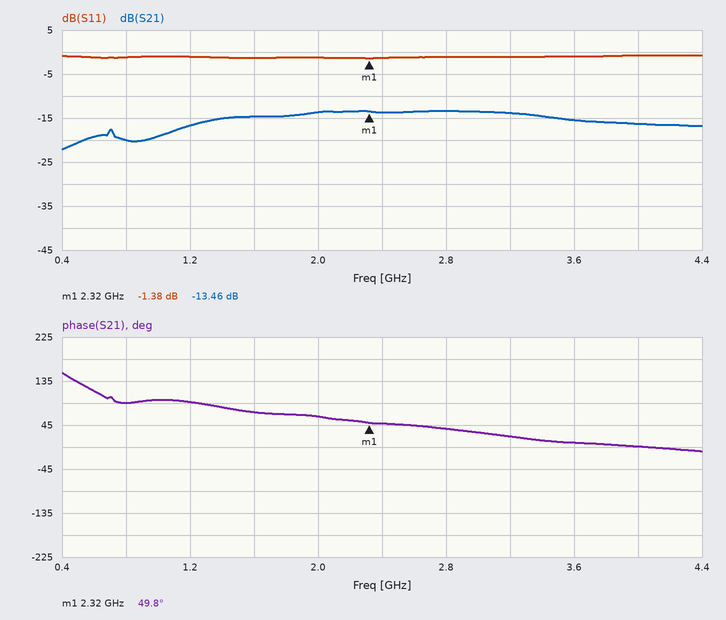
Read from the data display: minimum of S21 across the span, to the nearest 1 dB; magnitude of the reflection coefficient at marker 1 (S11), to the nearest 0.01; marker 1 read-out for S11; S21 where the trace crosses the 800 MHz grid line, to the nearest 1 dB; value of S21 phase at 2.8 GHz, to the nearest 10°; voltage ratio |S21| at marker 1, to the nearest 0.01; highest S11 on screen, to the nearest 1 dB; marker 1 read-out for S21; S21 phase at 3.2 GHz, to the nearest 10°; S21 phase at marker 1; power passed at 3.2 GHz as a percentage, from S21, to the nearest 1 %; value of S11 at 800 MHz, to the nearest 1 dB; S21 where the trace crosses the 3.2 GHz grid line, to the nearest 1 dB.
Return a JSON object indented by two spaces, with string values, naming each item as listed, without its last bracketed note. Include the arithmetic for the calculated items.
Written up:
{
  "minimum of S21 across the span, to the nearest 1 dB": "-22 dB",
  "magnitude of the reflection coefficient at marker 1 (S11), to the nearest 0.01": "10^(-1.38/20) ≈ 0.85",
  "marker 1 read-out for S11": "-1.38 dB",
  "S21 where the trace crosses the 800 MHz grid line, to the nearest 1 dB": "-20 dB",
  "value of S21 phase at 2.8 GHz, to the nearest 10°": "40°",
  "voltage ratio |S21| at marker 1, to the nearest 0.01": "10^(-13.46/20) ≈ 0.21",
  "highest S11 on screen, to the nearest 1 dB": "-1 dB",
  "marker 1 read-out for S21": "-13.46 dB",
  "S21 phase at 3.2 GHz, to the nearest 10°": "20°",
  "S21 phase at marker 1": "49.8°",
  "power passed at 3.2 GHz as a percentage, from S21, to the nearest 1 %": "10^(-14/10) ≈ 4 %",
  "value of S11 at 800 MHz, to the nearest 1 dB": "-1 dB",
  "S21 where the trace crosses the 3.2 GHz grid line, to the nearest 1 dB": "-14 dB"
}
